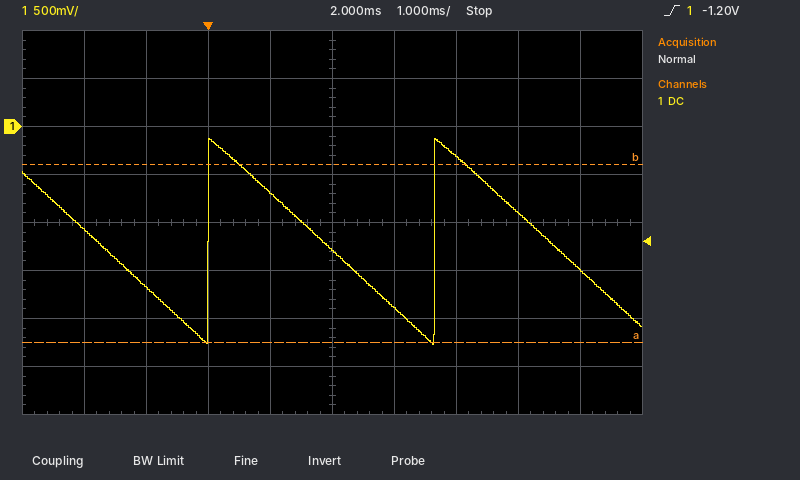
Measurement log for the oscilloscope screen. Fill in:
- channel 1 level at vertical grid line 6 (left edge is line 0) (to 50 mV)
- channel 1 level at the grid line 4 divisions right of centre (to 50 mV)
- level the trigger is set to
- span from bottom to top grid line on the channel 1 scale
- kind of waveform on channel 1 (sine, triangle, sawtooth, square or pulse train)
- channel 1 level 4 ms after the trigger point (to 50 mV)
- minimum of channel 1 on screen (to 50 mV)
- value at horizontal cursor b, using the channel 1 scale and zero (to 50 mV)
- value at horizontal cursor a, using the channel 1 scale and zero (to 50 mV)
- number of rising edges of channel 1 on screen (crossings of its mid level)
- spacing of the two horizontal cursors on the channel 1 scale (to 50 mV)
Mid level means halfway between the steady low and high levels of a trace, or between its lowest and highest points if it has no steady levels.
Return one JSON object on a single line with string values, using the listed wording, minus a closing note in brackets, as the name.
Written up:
{"channel 1 level at vertical grid line 6 (left edge is line 0)": "-1.90 V", "channel 1 level at the grid line 4 divisions right of centre": "-1.50 V", "level the trigger is set to": "-1.20 V", "span from bottom to top grid line on the channel 1 scale": "4 V", "kind of waveform on channel 1": "sawtooth", "channel 1 level 4 ms after the trigger point": "-300 mV", "minimum of channel 1 on screen": "-2.25 V", "value at horizontal cursor b, using the channel 1 scale and zero": "-400 mV", "value at horizontal cursor a, using the channel 1 scale and zero": "-2.25 V", "number of rising edges of channel 1 on screen": "2", "spacing of the two horizontal cursors on the channel 1 scale": "1.85 V"}
